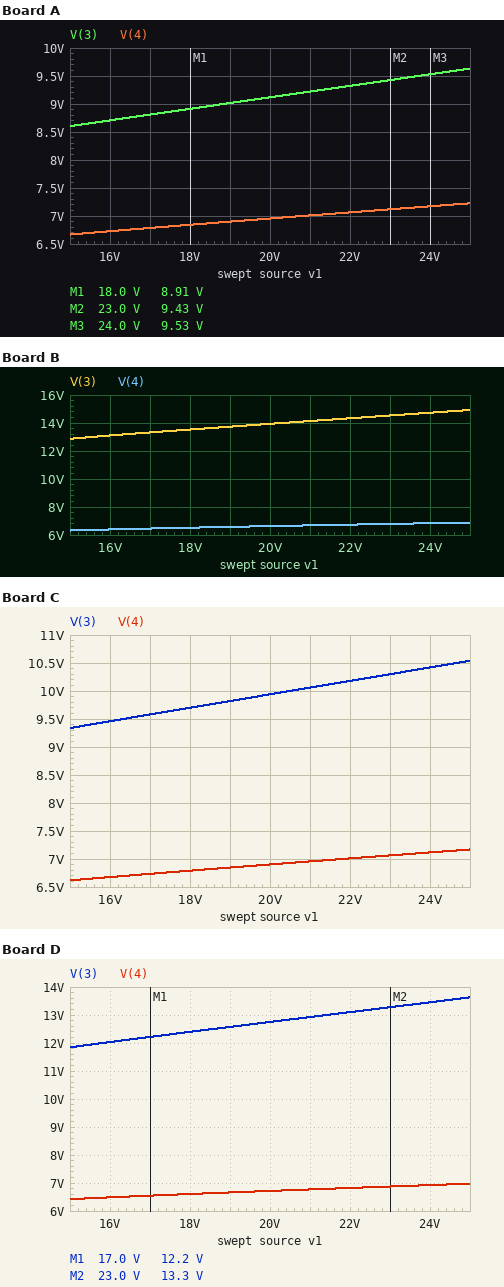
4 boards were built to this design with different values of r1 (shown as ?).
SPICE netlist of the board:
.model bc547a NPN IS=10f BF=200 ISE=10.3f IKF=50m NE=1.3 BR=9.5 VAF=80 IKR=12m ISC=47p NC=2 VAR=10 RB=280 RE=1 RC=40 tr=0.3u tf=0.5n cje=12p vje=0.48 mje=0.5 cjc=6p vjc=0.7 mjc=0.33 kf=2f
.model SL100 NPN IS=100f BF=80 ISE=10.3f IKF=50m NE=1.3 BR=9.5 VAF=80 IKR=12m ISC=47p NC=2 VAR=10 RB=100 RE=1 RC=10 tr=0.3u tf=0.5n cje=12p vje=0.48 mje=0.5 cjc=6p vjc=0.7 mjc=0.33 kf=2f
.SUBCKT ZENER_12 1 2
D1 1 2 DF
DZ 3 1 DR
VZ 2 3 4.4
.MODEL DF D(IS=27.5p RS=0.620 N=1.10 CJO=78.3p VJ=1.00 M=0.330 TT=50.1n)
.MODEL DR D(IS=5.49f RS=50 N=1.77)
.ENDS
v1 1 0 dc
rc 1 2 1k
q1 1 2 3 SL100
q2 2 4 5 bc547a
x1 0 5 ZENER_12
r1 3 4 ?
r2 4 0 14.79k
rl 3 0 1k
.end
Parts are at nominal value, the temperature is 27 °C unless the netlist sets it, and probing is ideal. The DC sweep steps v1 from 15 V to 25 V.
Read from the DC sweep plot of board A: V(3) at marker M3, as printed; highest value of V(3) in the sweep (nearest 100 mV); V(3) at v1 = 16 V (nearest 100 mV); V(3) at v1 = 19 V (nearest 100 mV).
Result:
9.53 V
9.6 V
8.7 V
9.0 V
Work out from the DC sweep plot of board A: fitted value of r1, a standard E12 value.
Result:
3.9 kΩ
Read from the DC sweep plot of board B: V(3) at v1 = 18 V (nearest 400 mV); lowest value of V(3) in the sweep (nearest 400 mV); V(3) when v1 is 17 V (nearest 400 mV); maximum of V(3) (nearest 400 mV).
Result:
13.6 V
12.8 V
13.2 V
14.8 V
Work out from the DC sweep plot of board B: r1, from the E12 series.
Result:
15 kΩ
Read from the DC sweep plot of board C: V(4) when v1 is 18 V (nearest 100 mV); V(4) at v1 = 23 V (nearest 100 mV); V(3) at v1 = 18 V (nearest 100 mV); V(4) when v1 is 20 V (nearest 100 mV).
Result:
6.8 V
7.1 V
9.7 V
6.9 V
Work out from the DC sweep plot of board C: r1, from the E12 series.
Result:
5.6 kΩ
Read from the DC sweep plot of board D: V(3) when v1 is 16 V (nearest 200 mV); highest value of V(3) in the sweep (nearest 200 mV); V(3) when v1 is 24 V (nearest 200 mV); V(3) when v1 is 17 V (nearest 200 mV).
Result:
12.0 V
13.6 V
13.4 V
12.2 V
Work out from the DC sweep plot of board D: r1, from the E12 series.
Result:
12 kΩ
